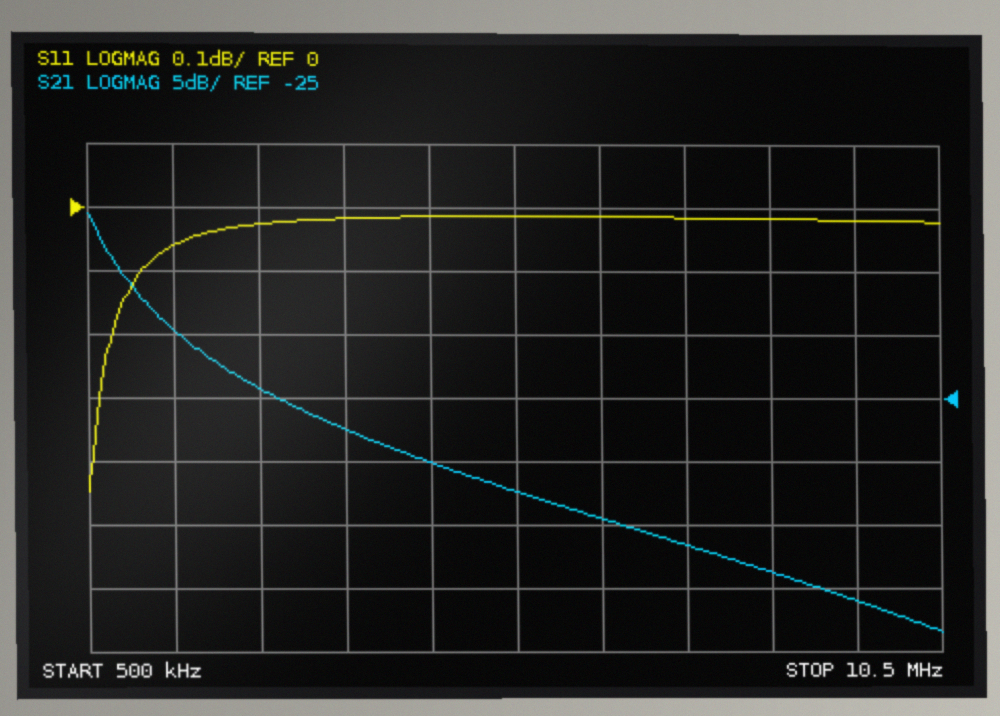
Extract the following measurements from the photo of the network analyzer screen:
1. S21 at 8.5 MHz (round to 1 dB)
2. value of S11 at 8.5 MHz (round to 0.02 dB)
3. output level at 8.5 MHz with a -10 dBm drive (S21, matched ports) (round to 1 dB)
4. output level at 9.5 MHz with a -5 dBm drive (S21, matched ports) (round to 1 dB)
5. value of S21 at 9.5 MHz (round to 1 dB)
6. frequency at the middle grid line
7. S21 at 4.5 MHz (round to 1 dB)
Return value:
-39 dB
-0.02 dB
-49 dBm
-46 dBm
-41 dB
5.5 MHz
-30 dB
